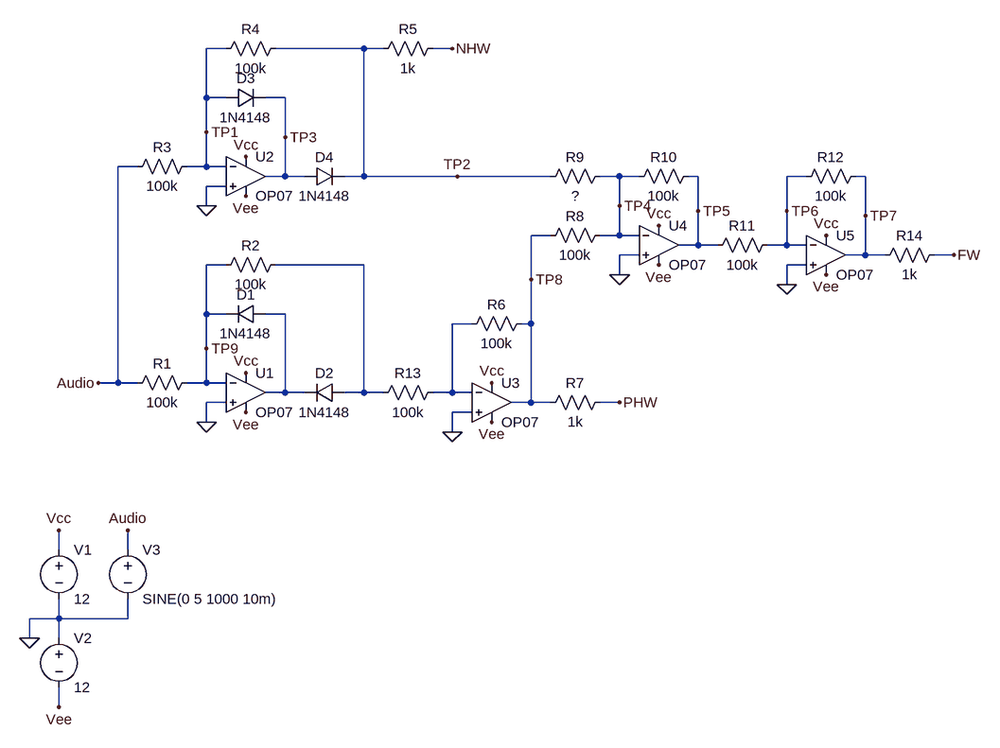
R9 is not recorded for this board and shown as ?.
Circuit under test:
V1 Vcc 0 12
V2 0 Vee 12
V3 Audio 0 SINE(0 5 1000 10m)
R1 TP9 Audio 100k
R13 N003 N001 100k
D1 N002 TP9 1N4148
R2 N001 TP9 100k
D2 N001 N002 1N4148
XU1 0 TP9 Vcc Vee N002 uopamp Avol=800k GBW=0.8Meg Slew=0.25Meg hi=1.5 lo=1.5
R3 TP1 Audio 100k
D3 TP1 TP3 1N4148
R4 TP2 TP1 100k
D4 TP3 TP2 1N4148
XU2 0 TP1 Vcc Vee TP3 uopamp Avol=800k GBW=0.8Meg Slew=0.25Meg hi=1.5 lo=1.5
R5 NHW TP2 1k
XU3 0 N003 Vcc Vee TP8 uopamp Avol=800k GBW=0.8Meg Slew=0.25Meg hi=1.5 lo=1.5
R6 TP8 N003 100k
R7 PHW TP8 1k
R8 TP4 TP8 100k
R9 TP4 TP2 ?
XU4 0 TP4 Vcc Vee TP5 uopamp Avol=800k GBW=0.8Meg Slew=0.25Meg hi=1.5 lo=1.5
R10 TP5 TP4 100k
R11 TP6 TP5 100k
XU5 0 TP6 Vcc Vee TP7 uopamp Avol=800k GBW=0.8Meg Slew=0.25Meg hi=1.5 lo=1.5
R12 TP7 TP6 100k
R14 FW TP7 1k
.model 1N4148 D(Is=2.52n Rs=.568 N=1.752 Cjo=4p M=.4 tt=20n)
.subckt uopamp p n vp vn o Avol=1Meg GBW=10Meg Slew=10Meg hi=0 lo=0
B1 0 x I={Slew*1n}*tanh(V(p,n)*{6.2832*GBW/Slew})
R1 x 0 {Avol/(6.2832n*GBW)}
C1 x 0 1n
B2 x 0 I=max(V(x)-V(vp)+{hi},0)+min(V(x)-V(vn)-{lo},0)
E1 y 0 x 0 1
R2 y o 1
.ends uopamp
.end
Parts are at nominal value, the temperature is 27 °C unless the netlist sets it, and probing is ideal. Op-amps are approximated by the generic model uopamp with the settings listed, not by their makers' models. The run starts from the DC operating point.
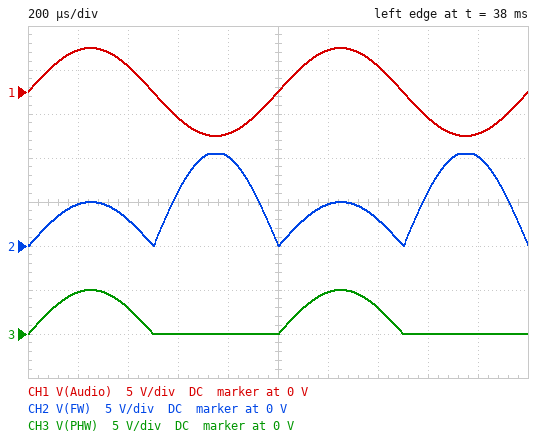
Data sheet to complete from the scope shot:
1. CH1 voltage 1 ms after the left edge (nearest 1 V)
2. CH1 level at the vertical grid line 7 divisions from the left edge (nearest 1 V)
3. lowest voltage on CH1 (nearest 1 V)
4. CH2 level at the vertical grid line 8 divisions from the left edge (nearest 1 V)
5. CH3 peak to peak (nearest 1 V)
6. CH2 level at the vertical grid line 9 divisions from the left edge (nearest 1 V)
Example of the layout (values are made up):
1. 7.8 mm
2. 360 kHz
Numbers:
1. 0 V
2. 3 V
3. -5 V
4. 6 V
5. 5 V
6. 10 V
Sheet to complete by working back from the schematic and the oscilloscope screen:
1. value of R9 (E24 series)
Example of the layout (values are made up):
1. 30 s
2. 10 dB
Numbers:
1. 47 kΩ
